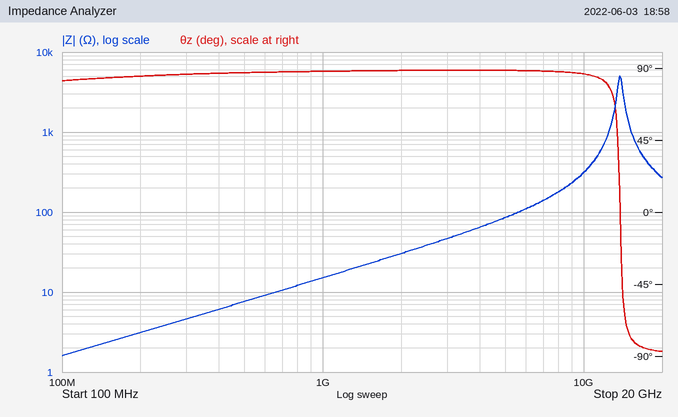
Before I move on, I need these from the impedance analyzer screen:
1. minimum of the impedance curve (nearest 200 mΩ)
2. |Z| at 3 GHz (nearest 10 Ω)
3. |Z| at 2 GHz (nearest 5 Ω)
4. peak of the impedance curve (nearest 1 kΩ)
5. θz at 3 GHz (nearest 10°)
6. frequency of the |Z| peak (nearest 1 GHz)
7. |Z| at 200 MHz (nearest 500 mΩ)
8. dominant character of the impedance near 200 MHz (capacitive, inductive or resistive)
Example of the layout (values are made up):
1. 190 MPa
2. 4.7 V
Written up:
1. 1.6 Ω
2. 50 Ω
3. 30 Ω
4. 5 kΩ
5. 90°
6. 14 GHz
7. 3.0 Ω
8. inductive
